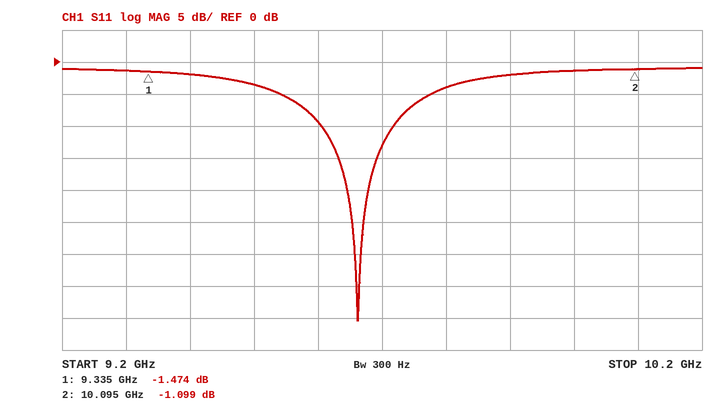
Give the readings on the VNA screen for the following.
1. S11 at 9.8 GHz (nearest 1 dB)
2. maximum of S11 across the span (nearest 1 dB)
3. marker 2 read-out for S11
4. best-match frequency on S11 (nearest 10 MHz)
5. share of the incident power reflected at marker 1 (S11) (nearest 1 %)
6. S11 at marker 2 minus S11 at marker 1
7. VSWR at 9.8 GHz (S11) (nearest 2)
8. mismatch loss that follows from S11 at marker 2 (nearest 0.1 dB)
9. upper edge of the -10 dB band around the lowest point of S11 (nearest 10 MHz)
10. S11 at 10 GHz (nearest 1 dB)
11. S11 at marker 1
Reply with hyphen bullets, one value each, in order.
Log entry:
- -4 dB
- -1 dB
- -1.099 dB
- 9.66 GHz
- 71 %
- 0.375 dB
- 4
- 6.5 dB
- 9.72 GHz
- -1 dB
- -1.474 dB
